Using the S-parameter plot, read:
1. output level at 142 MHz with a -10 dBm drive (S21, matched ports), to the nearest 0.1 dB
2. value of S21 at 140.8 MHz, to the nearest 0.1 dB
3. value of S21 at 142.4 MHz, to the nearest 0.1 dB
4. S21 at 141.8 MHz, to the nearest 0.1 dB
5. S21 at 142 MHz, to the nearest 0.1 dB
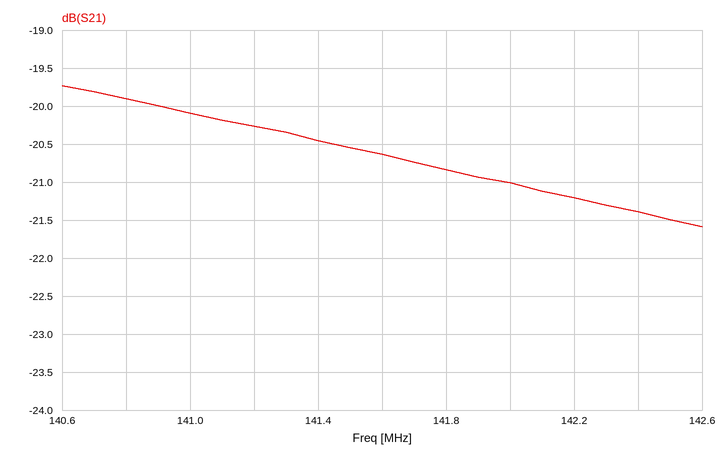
-31.0 dBm
-19.9 dB
-21.4 dB
-20.8 dB
-21.0 dB
